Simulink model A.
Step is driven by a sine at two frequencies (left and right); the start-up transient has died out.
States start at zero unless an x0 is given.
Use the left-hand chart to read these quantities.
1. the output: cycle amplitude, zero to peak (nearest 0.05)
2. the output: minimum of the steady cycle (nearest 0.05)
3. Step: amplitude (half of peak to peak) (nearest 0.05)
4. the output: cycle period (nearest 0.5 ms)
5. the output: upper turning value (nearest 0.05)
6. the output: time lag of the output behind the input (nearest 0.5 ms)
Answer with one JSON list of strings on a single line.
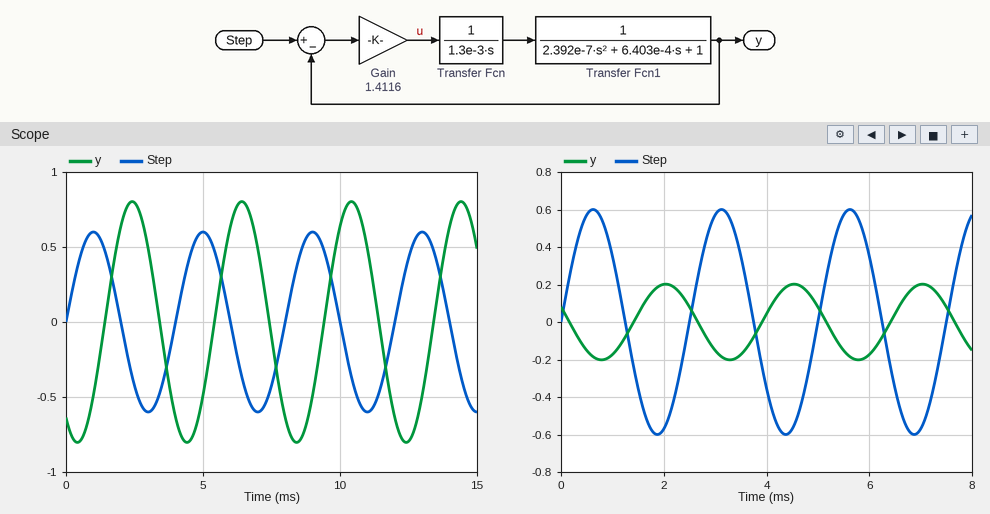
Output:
["0.80", "-0.80", "0.60", "4.0 ms", "0.80", "1.5 ms"]
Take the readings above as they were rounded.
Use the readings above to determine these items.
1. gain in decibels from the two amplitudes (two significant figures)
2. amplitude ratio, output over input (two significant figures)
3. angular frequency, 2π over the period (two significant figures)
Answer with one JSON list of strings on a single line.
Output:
["2.5 dB", "1.3", "1.6 rad/ms"]
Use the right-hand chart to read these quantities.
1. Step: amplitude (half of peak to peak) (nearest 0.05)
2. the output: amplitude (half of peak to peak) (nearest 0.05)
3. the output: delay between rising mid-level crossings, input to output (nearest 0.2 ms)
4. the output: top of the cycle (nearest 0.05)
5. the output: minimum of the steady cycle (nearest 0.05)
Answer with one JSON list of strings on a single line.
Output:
["0.60", "0.20", "1.4 ms", "0.20", "-0.20"]
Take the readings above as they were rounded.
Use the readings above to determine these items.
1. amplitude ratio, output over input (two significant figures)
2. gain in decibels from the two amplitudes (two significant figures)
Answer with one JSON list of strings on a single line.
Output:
["0.33", "-9.5 dB"]
